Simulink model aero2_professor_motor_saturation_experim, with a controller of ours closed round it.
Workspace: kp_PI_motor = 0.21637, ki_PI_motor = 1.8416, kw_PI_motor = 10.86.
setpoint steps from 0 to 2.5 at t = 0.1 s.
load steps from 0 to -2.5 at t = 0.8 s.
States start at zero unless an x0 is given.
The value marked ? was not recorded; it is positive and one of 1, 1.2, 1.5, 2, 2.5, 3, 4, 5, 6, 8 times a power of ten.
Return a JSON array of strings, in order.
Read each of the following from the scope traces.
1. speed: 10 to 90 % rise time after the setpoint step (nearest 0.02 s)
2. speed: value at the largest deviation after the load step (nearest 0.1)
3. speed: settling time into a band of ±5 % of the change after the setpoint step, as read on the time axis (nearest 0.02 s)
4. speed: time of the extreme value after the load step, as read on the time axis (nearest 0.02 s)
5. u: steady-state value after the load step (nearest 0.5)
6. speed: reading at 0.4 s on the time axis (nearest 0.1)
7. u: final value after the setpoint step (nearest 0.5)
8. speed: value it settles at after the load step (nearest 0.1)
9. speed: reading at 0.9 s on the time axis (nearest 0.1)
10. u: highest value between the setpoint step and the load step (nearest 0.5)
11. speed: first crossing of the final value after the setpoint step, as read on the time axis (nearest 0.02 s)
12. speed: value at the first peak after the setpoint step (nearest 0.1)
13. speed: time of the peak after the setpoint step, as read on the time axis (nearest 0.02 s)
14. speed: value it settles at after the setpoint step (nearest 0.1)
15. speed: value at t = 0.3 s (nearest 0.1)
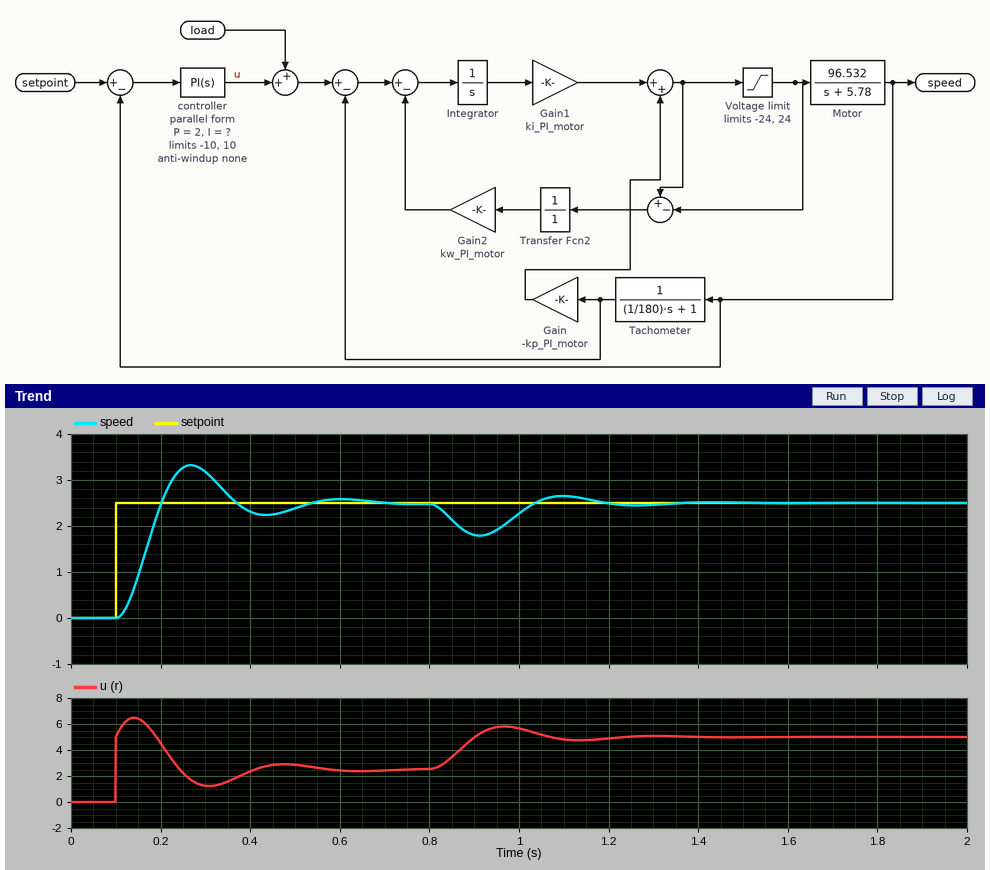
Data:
["0.06 s", "1.8", "0.50 s", "0.92 s", "5.0", "2.3", "2.5", "2.5", "1.8", "6.5", "0.20 s", "3.3", "0.26 s", "2.5", "3.2"]
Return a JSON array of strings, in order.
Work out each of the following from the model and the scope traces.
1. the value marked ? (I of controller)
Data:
["30"]
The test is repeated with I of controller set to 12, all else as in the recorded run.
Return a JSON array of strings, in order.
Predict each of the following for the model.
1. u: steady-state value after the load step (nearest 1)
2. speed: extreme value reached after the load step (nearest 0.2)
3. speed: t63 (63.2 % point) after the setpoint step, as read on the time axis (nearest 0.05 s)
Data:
["5", "1.6", "0.20 s"]
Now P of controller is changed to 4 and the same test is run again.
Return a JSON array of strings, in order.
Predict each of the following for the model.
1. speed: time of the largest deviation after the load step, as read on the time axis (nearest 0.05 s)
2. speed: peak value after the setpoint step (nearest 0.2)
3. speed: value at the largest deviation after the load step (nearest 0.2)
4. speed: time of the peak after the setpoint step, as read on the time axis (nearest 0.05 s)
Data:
["0.90 s", "3.2", "2.0", "0.20 s"]
